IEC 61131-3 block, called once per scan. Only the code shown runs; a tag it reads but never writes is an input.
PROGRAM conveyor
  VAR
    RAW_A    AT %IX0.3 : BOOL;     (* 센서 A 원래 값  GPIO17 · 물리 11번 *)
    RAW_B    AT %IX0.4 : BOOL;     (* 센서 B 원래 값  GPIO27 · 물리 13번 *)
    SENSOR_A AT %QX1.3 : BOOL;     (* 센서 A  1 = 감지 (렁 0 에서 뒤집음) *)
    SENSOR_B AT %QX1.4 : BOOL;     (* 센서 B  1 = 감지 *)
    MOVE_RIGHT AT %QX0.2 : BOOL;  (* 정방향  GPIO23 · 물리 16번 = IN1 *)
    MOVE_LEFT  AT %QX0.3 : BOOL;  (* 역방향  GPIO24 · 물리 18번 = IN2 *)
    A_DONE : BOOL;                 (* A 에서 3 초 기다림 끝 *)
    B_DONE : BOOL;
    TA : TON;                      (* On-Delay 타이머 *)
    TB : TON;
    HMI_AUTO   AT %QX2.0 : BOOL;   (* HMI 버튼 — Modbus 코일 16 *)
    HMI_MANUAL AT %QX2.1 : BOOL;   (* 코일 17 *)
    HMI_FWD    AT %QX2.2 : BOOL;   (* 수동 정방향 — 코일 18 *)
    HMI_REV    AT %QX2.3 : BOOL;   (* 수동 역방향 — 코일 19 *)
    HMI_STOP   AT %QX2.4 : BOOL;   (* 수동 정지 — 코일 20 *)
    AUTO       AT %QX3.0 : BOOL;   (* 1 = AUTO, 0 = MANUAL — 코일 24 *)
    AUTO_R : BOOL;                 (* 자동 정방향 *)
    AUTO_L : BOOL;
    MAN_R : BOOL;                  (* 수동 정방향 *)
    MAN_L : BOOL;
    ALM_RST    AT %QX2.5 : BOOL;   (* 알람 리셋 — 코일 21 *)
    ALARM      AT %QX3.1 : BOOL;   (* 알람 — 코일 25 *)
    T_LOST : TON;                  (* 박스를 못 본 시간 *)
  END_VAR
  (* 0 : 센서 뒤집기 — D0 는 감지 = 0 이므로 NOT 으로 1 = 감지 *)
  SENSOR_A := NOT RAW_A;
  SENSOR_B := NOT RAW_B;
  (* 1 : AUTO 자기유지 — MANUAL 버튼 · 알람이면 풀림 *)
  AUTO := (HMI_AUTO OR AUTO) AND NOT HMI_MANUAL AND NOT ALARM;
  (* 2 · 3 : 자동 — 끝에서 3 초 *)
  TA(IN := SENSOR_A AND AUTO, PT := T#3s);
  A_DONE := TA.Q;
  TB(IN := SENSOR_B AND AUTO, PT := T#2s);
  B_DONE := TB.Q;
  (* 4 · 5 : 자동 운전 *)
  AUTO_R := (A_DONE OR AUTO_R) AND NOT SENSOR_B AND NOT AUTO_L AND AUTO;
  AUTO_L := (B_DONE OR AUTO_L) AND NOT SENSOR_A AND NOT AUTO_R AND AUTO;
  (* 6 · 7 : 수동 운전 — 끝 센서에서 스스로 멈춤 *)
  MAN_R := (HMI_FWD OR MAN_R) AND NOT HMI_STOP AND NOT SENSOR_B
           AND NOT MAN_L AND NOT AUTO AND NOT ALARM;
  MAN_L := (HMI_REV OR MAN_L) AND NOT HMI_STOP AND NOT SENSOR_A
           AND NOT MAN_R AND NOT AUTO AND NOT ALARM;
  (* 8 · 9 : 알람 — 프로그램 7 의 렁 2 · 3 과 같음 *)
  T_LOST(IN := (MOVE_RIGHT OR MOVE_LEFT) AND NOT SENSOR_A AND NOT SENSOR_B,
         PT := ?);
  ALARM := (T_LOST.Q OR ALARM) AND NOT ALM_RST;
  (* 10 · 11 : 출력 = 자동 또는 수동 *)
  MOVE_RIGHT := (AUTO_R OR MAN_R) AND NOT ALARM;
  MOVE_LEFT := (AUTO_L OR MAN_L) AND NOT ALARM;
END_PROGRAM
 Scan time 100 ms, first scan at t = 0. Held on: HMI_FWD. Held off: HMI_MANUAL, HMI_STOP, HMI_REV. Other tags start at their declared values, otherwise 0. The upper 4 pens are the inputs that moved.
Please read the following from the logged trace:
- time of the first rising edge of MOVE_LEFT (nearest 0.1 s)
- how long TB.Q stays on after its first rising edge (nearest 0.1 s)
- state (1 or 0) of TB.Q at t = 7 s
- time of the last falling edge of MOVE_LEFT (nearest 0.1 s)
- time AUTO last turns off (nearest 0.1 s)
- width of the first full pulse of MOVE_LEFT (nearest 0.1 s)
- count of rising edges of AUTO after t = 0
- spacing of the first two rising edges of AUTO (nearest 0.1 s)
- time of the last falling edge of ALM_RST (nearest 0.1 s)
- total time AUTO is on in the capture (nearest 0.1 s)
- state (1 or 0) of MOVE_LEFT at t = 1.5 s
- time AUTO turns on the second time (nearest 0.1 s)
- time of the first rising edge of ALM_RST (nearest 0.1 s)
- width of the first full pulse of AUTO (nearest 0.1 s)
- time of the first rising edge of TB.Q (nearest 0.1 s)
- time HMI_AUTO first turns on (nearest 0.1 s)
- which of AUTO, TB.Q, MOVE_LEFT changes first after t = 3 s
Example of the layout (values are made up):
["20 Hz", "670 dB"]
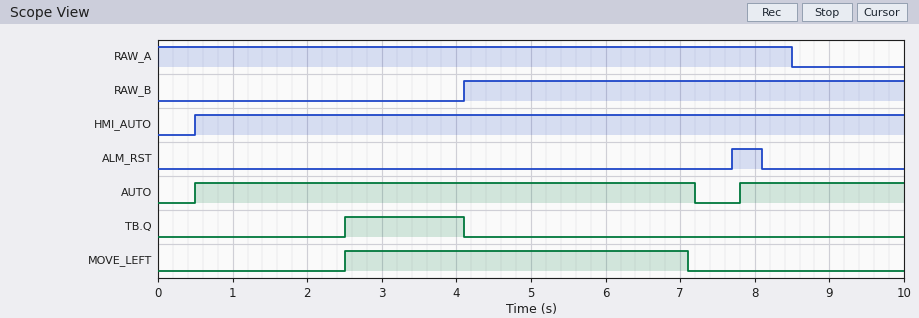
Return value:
["2.5 s", "1.6 s", "0", "7.1 s", "7.2 s", "4.6 s", "2", "7.3 s", "8.1 s", "8.9 s", "0", "7.8 s", "7.7 s", "6.7 s", "2.5 s", "0.5 s", "TB.Q"]
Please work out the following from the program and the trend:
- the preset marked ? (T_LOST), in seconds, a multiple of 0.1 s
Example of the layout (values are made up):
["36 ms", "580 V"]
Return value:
["3.0 s"]
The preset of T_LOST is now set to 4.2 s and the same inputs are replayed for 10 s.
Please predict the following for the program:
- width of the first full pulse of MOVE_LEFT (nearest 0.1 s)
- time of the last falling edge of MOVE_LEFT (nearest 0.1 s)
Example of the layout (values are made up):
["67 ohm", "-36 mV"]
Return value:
["5.8 s", "8.3 s"]
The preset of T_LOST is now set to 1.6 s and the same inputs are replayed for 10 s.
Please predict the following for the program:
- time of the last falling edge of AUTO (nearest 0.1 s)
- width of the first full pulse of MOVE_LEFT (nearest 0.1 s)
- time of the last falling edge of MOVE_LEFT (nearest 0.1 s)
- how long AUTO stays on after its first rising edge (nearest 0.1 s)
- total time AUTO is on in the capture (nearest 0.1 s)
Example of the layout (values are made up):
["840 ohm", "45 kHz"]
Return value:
["5.8 s", "3.2 s", "5.7 s", "5.3 s", "7.5 s"]
